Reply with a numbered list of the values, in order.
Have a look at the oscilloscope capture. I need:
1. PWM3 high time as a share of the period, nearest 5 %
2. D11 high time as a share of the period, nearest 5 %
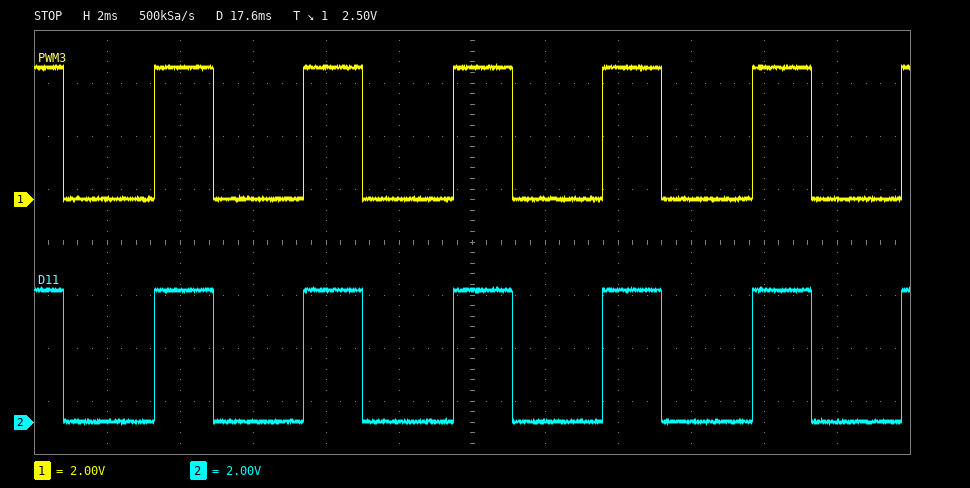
1. 40 %
2. 40 %
